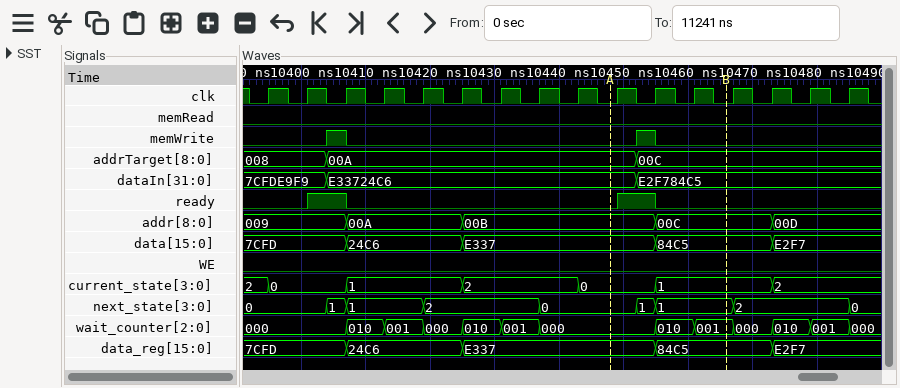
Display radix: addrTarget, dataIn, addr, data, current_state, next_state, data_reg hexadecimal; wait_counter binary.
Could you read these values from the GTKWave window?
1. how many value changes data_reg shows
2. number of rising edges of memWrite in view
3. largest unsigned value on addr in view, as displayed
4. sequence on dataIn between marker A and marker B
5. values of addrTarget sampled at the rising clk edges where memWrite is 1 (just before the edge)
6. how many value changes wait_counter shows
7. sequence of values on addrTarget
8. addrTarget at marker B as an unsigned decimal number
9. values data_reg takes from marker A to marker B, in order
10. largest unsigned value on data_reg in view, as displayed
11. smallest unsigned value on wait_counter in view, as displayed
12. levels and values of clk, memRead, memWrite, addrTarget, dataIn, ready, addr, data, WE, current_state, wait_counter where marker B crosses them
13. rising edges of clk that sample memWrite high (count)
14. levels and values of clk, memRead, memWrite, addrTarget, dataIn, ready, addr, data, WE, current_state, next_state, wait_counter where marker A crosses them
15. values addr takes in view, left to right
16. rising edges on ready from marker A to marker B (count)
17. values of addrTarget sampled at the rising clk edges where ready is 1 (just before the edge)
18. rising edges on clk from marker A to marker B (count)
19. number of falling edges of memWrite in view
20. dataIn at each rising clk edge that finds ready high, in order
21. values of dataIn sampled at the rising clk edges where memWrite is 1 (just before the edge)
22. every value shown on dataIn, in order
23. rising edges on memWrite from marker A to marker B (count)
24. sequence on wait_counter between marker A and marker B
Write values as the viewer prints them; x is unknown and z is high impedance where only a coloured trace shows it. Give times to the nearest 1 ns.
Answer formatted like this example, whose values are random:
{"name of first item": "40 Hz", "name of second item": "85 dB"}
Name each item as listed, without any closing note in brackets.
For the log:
{"how many value changes data_reg shows": "4", "number of rising edges of memWrite in view": "2", "largest unsigned value on addr in view, as displayed": "00D", "sequence on dataIn between marker A and marker B": "E33724C6, E2F784C5", "values of addrTarget sampled at the rising clk edges where memWrite is 1": "00A, 00C", "how many value changes wait_counter shows": "12", "sequence of values on addrTarget": "008, 00A, 00C", "addrTarget at marker B as an unsigned decimal number": "12", "values data_reg takes from marker A to marker B, in order": "E337, 84C5", "largest unsigned value on data_reg in view, as displayed": "E337", "smallest unsigned value on wait_counter in view, as displayed": "000", "levels and values of clk, memRead, memWrite, addrTarget, dataIn, ready, addr, data, WE, current_state, wait_counter where marker B crosses them": "clk=0, memRead=0, memWrite=0, addrTarget=00C, dataIn=E2F784C5, ready=0, addr=00C, data=84C5, WE=0, current_state=1, wait_counter=001", "rising edges of clk that sample memWrite high": "2", "levels and values of clk, memRead, memWrite, addrTarget, dataIn, ready, addr, data, WE, current_state, next_state, wait_counter where marker A crosses them": "clk=0, memRead=0, memWrite=0, addrTarget=00A, dataIn=E33724C6, ready=0, addr=00B, data=E337, WE=0, current_state=0, next_state=0, wait_counter=000", "values addr takes in view, left to right": "009, 00A, 00B, 00C, 00D", "rising edges on ready from marker A to marker B": "1", "values of addrTarget sampled at the rising clk edges where ready is 1": "00A, 00C", "rising edges on clk from marker A to marker B": "3", "number of falling edges of memWrite in view": "2", "dataIn at each rising clk edge that finds ready high, in order": "E33724C6, E2F784C5", "values of dataIn sampled at the rising clk edges where memWrite is 1": "E33724C6, E2F784C5", "every value shown on dataIn, in order": "7CFDE9F9, E33724C6, E2F784C5", "rising edges on memWrite from marker A to marker B": "1", "sequence on wait_counter between marker A and marker B": "000, 010, 001"}
